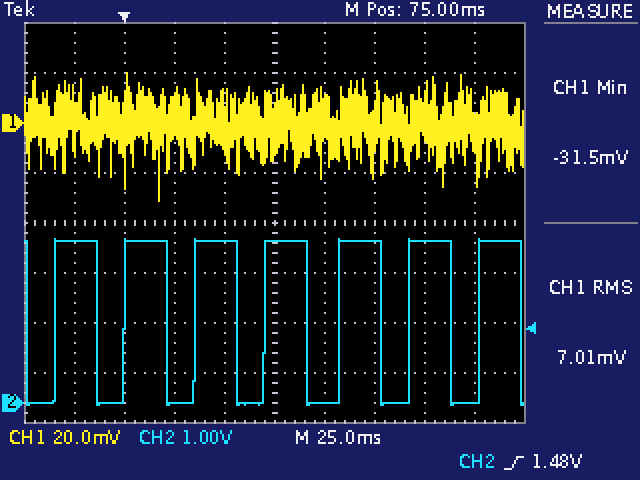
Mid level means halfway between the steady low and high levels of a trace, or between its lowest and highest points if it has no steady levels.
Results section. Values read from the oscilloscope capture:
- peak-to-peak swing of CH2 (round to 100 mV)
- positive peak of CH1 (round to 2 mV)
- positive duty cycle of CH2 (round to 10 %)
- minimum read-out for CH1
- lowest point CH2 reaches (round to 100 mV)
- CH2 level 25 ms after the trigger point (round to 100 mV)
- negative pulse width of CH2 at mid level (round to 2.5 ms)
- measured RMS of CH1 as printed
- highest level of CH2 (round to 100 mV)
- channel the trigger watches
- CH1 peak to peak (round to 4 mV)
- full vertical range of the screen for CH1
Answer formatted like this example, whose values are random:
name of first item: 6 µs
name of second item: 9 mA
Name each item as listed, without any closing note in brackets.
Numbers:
peak-to-peak swing of CH2: 3.3 V
positive peak of CH1: 20 mV
positive duty cycle of CH2: 60 %
minimum read-out for CH1: -31.5 mV
lowest point CH2 reaches: 0.0 V
CH2 level 25 ms after the trigger point: 0.0 V
negative pulse width of CH2 at mid level: 15.0 ms
measured RMS of CH1 as printed: 7.01 mV
highest level of CH2: 3.3 V
channel the trigger watches: CH2
CH1 peak to peak: 52 mV
full vertical range of the screen for CH1: 160 mV
